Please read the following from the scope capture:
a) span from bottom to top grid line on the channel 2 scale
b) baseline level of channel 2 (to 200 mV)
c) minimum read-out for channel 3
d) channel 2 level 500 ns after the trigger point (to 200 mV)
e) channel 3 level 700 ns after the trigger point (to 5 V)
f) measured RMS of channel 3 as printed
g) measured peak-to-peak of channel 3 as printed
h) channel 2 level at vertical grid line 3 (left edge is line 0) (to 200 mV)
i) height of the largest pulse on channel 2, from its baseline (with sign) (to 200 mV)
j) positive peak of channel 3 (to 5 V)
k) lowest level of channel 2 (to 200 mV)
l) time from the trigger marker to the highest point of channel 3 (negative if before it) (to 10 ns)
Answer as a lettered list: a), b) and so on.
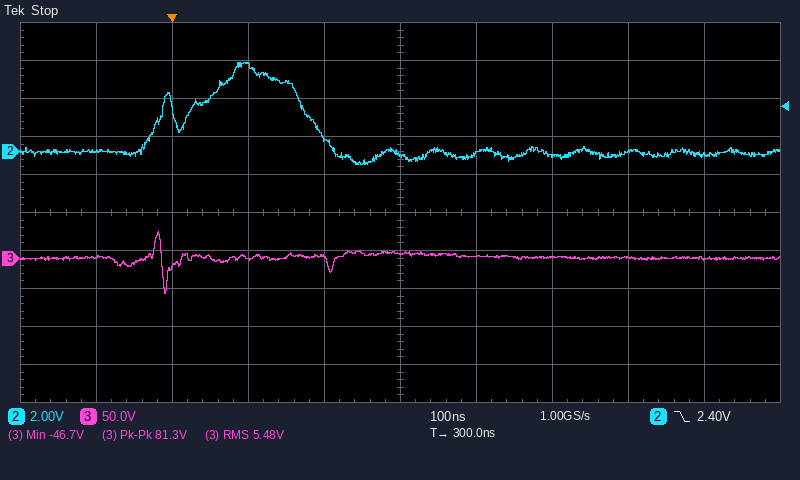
a) 20 V
b) 0.0 V
c) -46.7 V
d) -200 mV
e) 0 V
f) 5.48 V
g) 81.3 V
h) 4.6 V
i) +4.8 V
j) 35 V
k) -600 mV
l) -20 ns
